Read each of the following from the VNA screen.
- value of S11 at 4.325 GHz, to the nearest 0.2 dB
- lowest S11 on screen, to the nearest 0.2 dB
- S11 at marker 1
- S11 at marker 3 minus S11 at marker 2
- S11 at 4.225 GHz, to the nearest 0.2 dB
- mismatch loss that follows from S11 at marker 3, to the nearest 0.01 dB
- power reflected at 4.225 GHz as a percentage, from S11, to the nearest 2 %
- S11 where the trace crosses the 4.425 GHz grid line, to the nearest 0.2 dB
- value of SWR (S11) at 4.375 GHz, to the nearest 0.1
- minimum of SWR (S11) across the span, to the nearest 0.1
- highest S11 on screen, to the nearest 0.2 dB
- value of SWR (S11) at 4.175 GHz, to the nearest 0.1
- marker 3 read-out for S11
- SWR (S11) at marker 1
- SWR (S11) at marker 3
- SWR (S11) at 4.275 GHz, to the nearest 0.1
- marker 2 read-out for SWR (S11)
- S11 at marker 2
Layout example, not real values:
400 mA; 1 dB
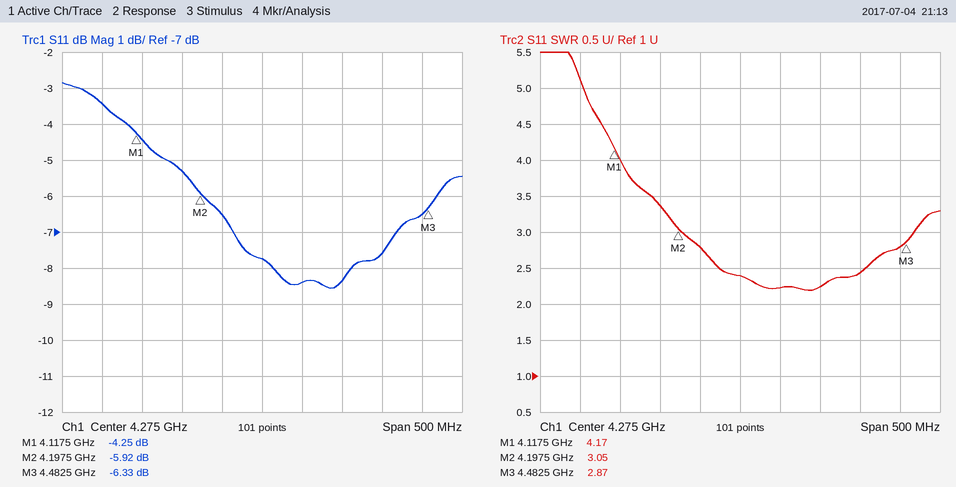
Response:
-8.4 dB; -8.6 dB; -4.25 dB; -0.41 dB; -6.6 dB; 1.15 dB; 22 %; -7.6 dB; 2.2; 2.2; -2.8 dB; 3.4; -6.33 dB; 4.17; 2.87; 2.4; 3.05; -5.92 dB
